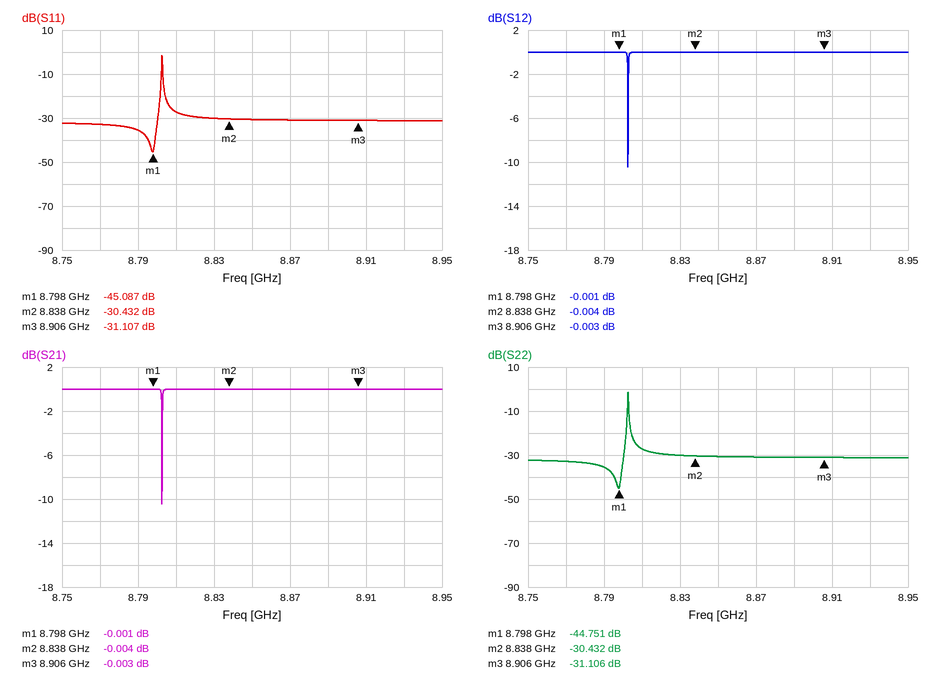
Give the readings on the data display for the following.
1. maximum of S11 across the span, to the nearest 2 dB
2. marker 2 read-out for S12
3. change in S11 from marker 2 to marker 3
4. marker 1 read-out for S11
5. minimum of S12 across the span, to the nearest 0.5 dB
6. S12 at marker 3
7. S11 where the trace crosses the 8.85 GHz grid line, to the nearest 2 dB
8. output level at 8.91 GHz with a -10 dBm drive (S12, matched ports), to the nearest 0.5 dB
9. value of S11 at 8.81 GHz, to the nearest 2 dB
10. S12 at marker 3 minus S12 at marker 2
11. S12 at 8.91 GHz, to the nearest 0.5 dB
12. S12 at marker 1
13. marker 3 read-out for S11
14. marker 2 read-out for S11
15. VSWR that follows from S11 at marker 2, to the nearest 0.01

-2 dB
-0.004 dB
-0.675 dB
-45.087 dB
-10.5 dB
-0.003 dB
-30 dB
-10.0 dBm
-28 dB
0.001 dB
0.0 dB
-0.001 dB
-31.107 dB
-30.432 dB
1.06
